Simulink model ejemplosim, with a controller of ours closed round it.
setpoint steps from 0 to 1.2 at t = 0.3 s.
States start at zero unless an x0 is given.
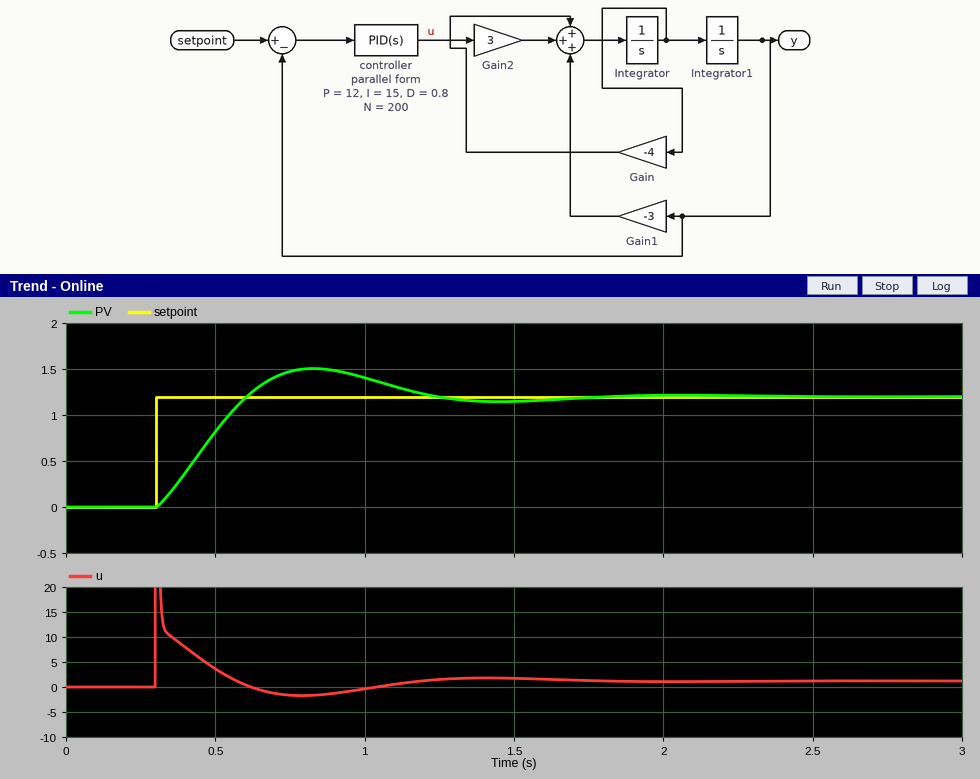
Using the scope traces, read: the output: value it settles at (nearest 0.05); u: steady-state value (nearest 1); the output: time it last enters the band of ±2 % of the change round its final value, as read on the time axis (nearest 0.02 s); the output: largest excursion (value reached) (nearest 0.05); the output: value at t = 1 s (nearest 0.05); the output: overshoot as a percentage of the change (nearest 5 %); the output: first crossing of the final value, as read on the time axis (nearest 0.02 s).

1.20
1
1.68 s
1.50
1.40
25 %
0.60 s
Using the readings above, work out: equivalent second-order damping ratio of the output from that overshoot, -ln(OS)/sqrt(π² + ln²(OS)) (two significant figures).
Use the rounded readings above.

0.40
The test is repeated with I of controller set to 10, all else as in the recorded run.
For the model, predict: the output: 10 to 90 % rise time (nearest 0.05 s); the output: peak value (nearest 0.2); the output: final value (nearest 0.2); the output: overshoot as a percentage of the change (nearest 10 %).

0.25 s
1.4
1.2
20 %
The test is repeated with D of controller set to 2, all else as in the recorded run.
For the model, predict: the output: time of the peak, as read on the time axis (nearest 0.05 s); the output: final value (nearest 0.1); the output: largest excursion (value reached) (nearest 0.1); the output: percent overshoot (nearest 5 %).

0.85 s
1.2
1.3
10 %
